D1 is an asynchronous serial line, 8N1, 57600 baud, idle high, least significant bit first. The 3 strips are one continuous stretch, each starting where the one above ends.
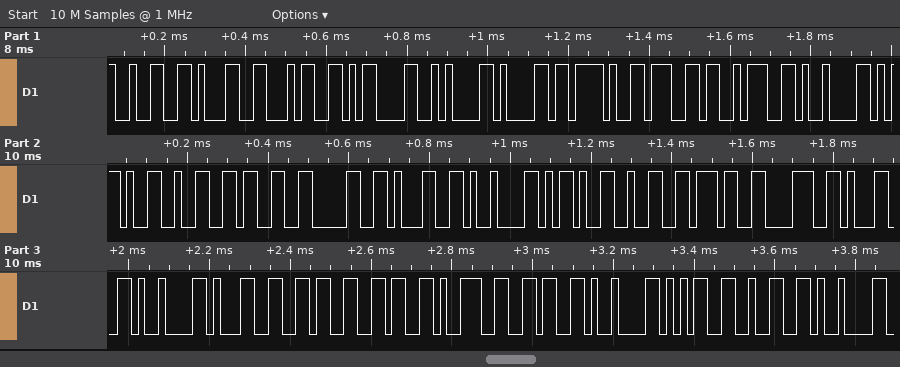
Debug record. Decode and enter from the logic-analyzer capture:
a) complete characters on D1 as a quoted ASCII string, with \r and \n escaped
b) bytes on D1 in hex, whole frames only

"214\r\na/g:\t-2301\t-2781\t16696\t52\t"
32 31 34 0D 0A 61 2F 67 3A 09 2D 32 33 30 31 09 2D 32 37 38 31 09 31 36 36 39 36 09 35 32 09
